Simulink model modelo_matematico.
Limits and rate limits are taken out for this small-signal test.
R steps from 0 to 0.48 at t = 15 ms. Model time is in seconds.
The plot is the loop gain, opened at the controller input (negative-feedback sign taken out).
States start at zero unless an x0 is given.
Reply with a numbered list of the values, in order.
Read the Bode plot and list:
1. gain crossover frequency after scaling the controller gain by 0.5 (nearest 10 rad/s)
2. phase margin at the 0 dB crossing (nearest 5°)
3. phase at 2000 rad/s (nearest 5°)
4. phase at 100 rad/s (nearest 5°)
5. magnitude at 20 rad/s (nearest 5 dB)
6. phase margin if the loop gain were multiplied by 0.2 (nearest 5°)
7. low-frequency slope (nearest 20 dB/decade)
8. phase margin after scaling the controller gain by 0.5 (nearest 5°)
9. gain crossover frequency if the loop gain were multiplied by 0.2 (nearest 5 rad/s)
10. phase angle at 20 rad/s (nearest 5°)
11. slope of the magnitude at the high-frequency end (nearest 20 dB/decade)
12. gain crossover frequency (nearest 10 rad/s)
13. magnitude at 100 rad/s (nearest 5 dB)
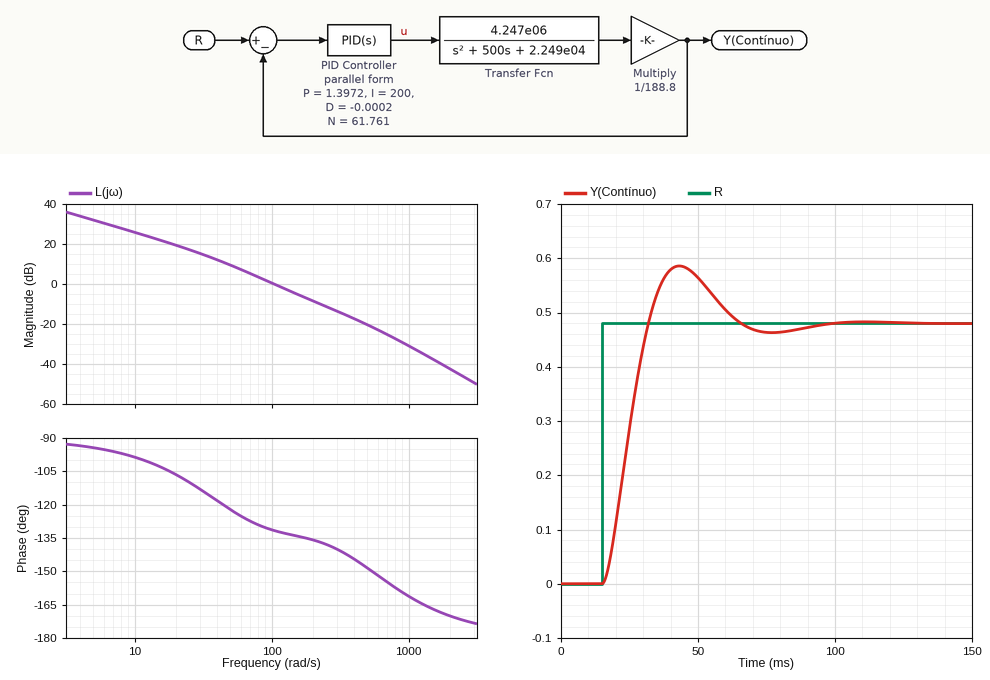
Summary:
1. 70 rad/s
2. 50°
3. -170°
4. -130°
5. 20 dB
6. 65°
7. -20 dB/decade
8. 55°
9. 35 rad/s
10. -105°
11. -40 dB/decade
12. 100 rad/s
13. 0 dB
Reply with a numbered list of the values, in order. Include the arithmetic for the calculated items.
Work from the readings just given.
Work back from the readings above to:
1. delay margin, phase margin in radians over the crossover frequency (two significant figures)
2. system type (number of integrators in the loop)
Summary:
1. 50 × π / 180 / 100 = 0.0087 s
2. 1
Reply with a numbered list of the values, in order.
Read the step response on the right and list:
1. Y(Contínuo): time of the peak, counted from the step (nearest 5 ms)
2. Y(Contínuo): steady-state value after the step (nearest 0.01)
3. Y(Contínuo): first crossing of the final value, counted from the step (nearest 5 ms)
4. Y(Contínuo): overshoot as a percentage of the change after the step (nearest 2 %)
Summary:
1. 30 ms
2. 0.48
3. 15 ms
4. 22 %
